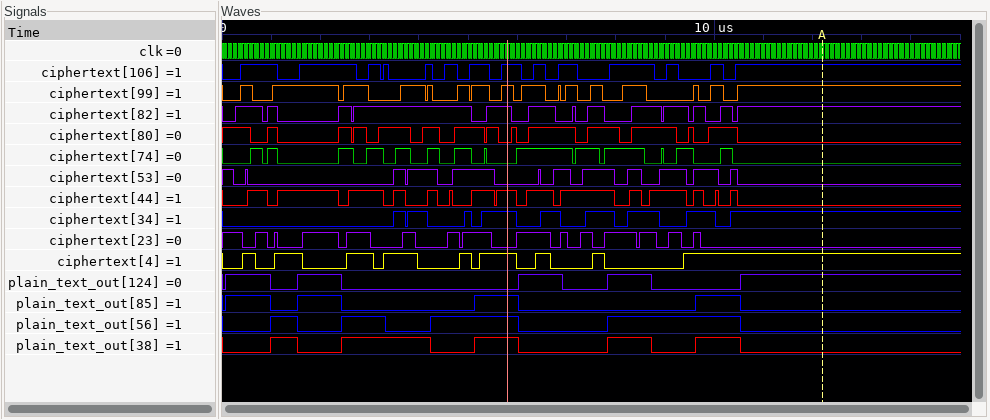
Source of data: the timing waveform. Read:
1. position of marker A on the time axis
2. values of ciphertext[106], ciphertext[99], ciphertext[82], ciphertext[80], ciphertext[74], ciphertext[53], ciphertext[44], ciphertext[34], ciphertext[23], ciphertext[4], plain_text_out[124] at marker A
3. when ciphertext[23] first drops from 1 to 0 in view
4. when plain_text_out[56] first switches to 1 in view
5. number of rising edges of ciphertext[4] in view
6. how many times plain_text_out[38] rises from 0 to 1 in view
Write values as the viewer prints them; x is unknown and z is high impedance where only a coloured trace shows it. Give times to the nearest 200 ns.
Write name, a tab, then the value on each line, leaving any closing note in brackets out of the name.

position of marker A on the time axis	12200 ns
values of ciphertext[106], ciphertext[99], ciphertext[82], ciphertext[80], ciphertext[74], ciphertext[53], ciphertext[44], ciphertext[34], ciphertext[23], ciphertext[4], plain_text_out[124] at marker A	ciphertext[106]=1, ciphertext[99]=1, ciphertext[82]=1, ciphertext[80]=0, ciphertext[74]=0, ciphertext[53]=0, ciphertext[44]=0, ciphertext[34]=1, ciphertext[23]=0, ciphertext[4]=1, plain_text_out[124]=1
when ciphertext[23] first drops from 1 to 0 in view	400 ns
when plain_text_out[56] first switches to 1 in view	1000 ns
number of rising edges of ciphertext[4] in view	9
how many times plain_text_out[38] rises from 0 to 1 in view	5
